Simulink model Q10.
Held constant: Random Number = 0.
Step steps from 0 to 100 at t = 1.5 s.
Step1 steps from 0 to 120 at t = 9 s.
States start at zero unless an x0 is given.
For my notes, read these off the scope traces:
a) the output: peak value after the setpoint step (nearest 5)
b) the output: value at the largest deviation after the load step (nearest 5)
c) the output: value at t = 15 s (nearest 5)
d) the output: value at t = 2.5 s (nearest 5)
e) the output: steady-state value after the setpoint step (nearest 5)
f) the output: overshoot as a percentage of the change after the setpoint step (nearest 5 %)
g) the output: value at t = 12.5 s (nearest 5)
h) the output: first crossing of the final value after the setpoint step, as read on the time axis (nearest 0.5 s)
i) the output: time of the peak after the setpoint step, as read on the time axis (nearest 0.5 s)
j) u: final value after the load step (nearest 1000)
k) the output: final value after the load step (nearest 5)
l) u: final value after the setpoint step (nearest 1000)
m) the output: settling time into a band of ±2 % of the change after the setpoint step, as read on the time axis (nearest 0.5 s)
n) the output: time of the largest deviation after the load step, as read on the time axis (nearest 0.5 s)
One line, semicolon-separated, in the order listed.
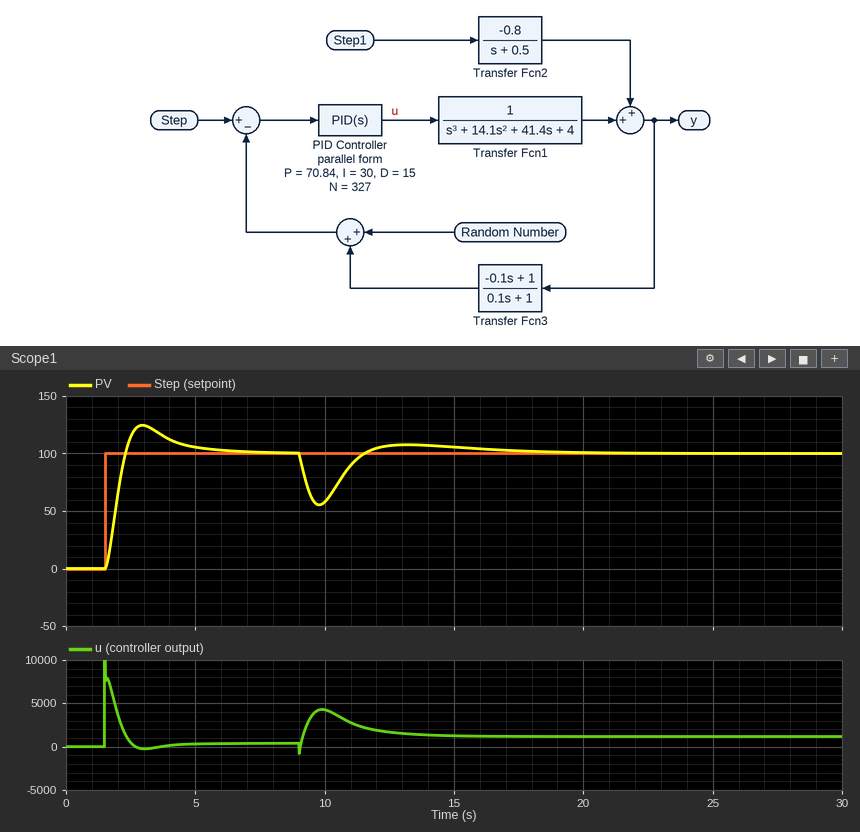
125; 55; 105; 115; 100; 25 %; 105; 2.5 s; 3.0 s; 1000; 100; 0; 6.5 s; 10.0 s
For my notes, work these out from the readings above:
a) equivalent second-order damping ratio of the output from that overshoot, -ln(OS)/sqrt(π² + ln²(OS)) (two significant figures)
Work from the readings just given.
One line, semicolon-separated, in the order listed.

0.40
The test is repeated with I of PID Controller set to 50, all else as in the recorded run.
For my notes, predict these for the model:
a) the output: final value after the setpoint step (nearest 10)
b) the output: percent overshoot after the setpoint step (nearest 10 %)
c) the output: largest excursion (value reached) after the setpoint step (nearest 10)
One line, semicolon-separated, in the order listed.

100; 40 %; 140
